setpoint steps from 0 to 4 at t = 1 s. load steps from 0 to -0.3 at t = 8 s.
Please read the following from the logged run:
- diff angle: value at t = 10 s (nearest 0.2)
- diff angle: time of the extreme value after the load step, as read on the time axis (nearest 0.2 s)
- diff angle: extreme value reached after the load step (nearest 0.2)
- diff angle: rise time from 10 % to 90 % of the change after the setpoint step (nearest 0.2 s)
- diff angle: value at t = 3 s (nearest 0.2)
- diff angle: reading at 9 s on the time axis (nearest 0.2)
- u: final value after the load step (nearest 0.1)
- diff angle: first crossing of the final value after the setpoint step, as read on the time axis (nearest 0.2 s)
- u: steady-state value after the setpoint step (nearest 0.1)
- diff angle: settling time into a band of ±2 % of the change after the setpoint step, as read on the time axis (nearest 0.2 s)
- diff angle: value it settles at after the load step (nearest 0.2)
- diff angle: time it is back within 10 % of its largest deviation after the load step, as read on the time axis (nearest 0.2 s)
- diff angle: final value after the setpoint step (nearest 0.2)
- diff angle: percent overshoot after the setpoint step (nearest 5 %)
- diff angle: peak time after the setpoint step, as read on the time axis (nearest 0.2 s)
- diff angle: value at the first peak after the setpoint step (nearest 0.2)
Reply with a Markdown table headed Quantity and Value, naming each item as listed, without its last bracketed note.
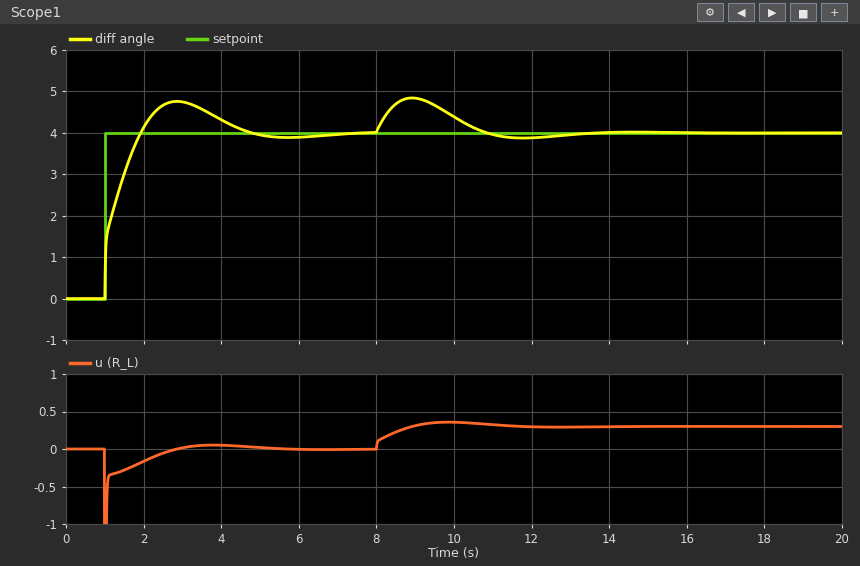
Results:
| Quantity | Value |
|---|---|
| diff angle: value at t = 10 s | 4.4 |
| diff angle: time of the extreme value after the load step, as read on the time axis | 9.0 s |
| diff angle: extreme value reached after the load step | 4.8 |
| diff angle: rise time from 10 % to 90 % of the change after the setpoint step | 0.8 s |
| diff angle: value at t = 3 s | 4.8 |
| diff angle: reading at 9 s on the time axis | 4.8 |
| u: final value after the load step | 0.3 |
| diff angle: first crossing of the final value after the setpoint step, as read on the time axis | 2.0 s |
| u: steady-state value after the setpoint step | 0.0 |
| diff angle: settling time into a band of ±2 % of the change after the setpoint step, as read on the time axis | 6.4 s |
| diff angle: value it settles at after the load step | 4.0 |
| diff angle: time it is back within 10 % of its largest deviation after the load step, as read on the time axis | 12.6 s |
| diff angle: final value after the setpoint step | 4.0 |
| diff angle: percent overshoot after the setpoint step | 20 % |
| diff angle: peak time after the setpoint step, as read on the time axis | 2.8 s |
| diff angle: value at the first peak after the setpoint step | 4.8 |
